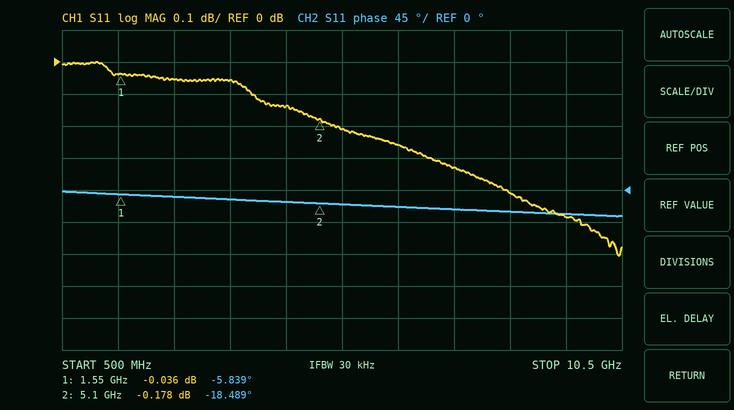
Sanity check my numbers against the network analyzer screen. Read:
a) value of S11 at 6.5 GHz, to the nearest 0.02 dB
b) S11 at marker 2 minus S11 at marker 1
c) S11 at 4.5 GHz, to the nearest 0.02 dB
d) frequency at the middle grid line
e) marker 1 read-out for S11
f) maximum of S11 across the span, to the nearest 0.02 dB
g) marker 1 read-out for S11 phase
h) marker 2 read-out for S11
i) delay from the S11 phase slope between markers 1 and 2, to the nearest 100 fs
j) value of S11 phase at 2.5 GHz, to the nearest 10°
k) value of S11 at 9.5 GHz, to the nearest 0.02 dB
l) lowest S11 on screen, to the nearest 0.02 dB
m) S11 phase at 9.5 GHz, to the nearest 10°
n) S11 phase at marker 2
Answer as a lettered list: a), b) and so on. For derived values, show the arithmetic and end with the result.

a) -0.26 dB
b) -0.178 − (-0.036) = -0.142 dB
c) -0.14 dB
d) 5.5 GHz
e) -0.036 dB
f) 0.00 dB
g) -5.839°
h) -0.178 dB
i) −(-18.489° − (-5.839°))/(360° × 3.55 GHz) ≈ 9.9 ps
j) -10°
k) -0.48 dB
l) -0.60 dB
m) -30°
n) -18.489°
